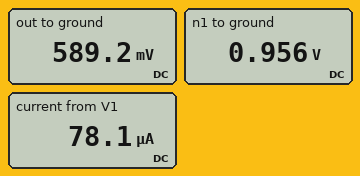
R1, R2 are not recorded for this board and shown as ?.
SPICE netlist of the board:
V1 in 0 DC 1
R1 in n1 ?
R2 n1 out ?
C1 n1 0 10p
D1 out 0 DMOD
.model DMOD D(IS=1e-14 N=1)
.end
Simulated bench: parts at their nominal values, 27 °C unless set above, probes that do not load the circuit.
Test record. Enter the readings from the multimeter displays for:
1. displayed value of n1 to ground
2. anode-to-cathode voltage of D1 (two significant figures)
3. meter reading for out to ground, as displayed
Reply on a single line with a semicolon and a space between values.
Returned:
0.956 V; 590 mV; 589.2 mV
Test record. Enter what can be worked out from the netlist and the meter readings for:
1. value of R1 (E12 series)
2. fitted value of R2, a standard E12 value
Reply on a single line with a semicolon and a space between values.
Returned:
560 Ω; 4.7 kΩ
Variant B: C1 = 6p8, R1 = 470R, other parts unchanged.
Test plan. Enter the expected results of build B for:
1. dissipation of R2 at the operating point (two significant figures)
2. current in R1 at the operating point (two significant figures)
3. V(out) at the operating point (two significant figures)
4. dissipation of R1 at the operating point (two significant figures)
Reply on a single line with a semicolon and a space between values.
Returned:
30 µW; 79 µA; 590 mV; 3.0 µW
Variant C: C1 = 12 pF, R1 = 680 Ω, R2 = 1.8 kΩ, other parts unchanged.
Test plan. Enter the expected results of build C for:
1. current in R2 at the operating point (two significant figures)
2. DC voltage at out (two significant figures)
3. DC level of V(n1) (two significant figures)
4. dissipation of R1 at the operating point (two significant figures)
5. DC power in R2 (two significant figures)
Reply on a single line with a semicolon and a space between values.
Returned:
160 µA; 610 mV; 890 mV; 17 µW; 45 µW
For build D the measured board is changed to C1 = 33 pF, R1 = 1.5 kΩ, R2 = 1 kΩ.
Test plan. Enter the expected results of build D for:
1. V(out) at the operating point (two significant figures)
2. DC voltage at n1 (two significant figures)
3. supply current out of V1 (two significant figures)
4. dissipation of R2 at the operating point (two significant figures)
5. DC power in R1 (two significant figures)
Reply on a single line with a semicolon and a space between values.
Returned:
610 mV; 760 mV; 160 µA; 25 µW; 37 µW
